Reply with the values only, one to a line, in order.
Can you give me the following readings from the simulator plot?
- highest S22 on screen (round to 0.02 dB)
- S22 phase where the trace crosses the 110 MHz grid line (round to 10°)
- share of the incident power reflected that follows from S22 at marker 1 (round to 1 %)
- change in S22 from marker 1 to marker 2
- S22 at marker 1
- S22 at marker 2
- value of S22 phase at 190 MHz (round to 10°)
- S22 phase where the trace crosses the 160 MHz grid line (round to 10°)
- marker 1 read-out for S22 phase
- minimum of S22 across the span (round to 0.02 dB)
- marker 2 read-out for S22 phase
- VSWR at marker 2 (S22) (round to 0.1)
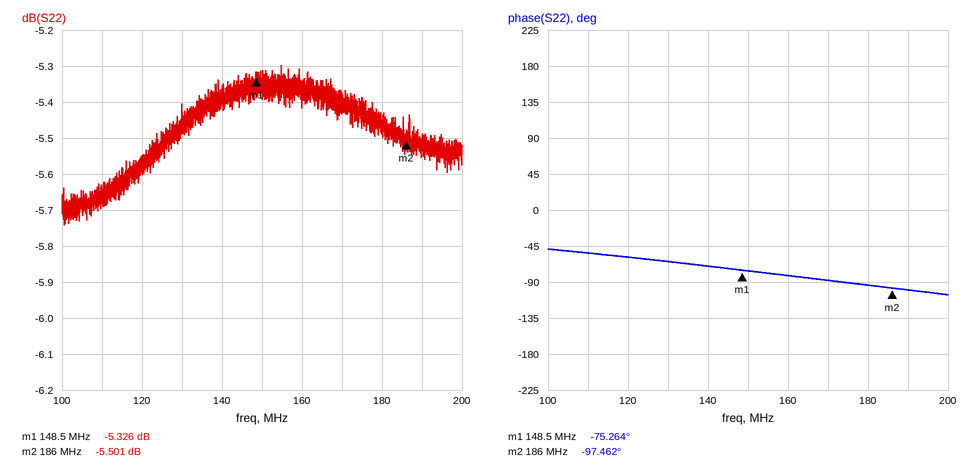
-5.30 dB
-50°
29 %
-0.175 dB
-5.326 dB
-5.501 dB
-100°
-80°
-75.264°
-5.74 dB
-97.462°
3.3
